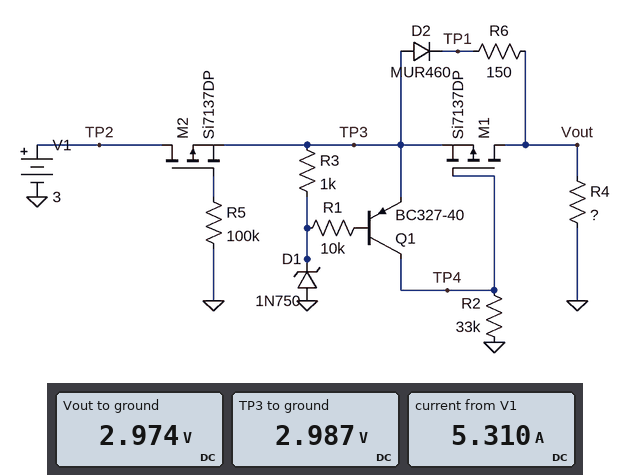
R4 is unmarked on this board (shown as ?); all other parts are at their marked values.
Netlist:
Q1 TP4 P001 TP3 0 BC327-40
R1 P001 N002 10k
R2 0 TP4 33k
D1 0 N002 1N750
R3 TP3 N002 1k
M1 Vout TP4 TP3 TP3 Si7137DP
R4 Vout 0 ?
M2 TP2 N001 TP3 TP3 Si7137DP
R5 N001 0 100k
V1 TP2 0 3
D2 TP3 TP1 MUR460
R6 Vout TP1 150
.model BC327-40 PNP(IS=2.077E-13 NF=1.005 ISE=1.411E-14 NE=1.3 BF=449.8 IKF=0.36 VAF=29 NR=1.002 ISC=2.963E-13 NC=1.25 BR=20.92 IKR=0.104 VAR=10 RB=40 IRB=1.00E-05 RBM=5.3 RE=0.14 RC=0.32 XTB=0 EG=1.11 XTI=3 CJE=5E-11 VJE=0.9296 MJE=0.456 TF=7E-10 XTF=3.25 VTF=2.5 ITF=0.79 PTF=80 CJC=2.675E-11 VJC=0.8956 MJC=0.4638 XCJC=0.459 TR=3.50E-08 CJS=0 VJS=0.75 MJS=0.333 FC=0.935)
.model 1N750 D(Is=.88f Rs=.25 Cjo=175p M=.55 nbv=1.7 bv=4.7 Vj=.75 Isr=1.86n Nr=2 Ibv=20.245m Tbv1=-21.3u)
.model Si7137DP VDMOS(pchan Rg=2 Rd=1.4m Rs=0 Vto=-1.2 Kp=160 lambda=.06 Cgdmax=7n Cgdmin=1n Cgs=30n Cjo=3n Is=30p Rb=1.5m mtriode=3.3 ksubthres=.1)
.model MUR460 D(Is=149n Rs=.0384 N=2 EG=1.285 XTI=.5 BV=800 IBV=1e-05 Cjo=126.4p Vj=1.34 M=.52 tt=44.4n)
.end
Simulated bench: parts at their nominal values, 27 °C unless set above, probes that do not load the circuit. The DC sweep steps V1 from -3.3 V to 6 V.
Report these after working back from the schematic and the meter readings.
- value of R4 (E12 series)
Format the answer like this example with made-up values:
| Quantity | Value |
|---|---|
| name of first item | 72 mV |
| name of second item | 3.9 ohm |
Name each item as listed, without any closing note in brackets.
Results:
| Quantity | Value |
|---|---|
| value of R4 | 0.56 Ω |
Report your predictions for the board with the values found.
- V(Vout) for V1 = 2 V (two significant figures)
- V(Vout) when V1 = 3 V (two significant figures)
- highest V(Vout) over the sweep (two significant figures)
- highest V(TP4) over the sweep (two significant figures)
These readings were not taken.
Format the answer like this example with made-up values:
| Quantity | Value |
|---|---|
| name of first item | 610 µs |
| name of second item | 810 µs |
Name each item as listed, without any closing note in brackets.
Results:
| Quantity | Value |
|---|---|
| V(Vout) for V1 = 2 V | 2.0 V |
| V(Vout) when V1 = 3 V | 3.0 V |
| highest V(Vout) over the sweep | 5.0 V |
| highest V(TP4) over the sweep | 6.0 V |
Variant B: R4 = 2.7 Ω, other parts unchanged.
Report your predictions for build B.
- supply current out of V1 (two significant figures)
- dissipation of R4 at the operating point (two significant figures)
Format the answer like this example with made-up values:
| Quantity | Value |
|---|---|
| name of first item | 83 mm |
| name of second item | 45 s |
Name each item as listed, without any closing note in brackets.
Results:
| Quantity | Value |
|---|---|
| supply current out of V1 | 1.1 A |
| dissipation of R4 at the operating point | 3.3 W |
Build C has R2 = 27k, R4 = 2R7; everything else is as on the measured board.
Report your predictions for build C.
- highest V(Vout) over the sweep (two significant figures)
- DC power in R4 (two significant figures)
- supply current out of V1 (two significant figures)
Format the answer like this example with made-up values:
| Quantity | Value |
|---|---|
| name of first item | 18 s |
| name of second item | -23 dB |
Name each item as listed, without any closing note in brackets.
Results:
| Quantity | Value |
|---|---|
| highest V(Vout) over the sweep | 5.1 V |
| DC power in R4 | 3.3 W |
| supply current out of V1 | 1.1 A |
